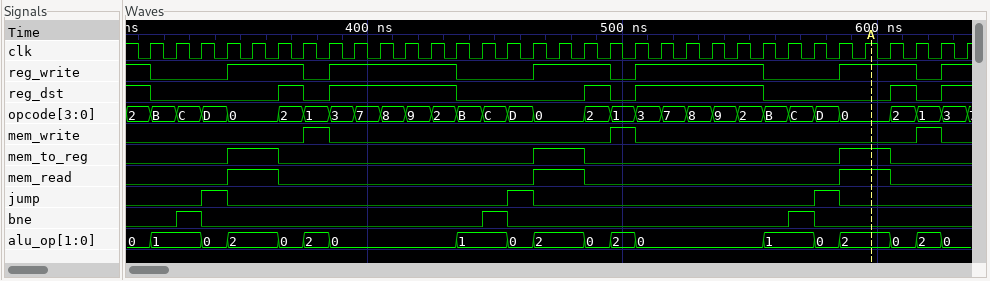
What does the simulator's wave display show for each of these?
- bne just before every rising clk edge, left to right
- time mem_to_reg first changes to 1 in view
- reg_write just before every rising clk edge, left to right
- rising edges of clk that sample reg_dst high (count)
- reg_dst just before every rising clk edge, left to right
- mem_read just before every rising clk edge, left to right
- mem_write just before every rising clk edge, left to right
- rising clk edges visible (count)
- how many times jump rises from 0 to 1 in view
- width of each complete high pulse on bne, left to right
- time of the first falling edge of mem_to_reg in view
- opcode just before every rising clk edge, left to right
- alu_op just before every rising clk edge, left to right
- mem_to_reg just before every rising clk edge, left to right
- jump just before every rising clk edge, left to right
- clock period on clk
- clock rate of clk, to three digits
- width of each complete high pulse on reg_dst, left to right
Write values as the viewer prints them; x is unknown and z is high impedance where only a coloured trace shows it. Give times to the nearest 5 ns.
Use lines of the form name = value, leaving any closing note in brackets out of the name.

bne just before every rising clk edge, left to right = 0 0 1 0 0 0 0 0 0 0 0 0 0 0 1 0 0 0 0 0 0 0 0 0 0 0 1 0 0 0 0 0 0
time mem_to_reg first changes to 1 in view = 345 ns
reg_write just before every rising clk edge, left to right = 1 0 0 0 1 1 1 0 1 1 1 1 1 0 0 0 1 1 1 0 1 1 1 1 1 0 0 0 1 1 1 0 1
rising edges of clk that sample reg_dst high = 15
reg_dst just before every rising clk edge, left to right = 1 0 0 0 0 0 1 0 1 1 1 1 1 0 0 0 0 0 1 0 1 1 1 1 1 0 0 0 0 0 1 0 1
mem_read just before every rising clk edge, left to right = 0 0 0 0 1 1 0 0 0 0 0 0 0 0 0 0 1 1 0 0 0 0 0 0 0 0 0 0 1 1 0 0 0
mem_write just before every rising clk edge, left to right = 0 0 0 0 0 0 0 1 0 0 0 0 0 0 0 0 0 0 0 1 0 0 0 0 0 0 0 0 0 0 0 1 0
rising clk edges visible = 33
how many times jump rises from 0 to 1 in view = 3
width of each complete high pulse on bne, left to right = 10 ns, 10 ns, 10 ns
time of the first falling edge of mem_to_reg in view = 365 ns
opcode just before every rising clk edge, left to right = 2, B, C, D, 0, 0, 2, 1, 3, 7, 8, 9, 2, B, C, D, 0, 0, 2, 1, 3, 7, 8, 9, 2, B, C, D, 0, 0, 2, 1, 3
alu_op just before every rising clk edge, left to right = 0, 1, 1, 0, 2, 2, 0, 2, 0, 0, 0, 0, 0, 1, 1, 0, 2, 2, 0, 2, 0, 0, 0, 0, 0, 1, 1, 0, 2, 2, 0, 2, 0
mem_to_reg just before every rising clk edge, left to right = 0 0 0 0 1 1 0 0 0 0 0 0 0 0 0 0 1 1 0 0 0 0 0 0 0 0 0 0 1 1 0 0 0
jump just before every rising clk edge, left to right = 0 0 0 1 0 0 0 0 0 0 0 0 0 0 0 1 0 0 0 0 0 0 0 0 0 0 0 1 0 0 0 0 0
clock period on clk = 10 ns
clock rate of clk, to three digits = 100 MHz
width of each complete high pulse on reg_dst, left to right = 10 ns, 50 ns, 10 ns, 50 ns, 10 ns
